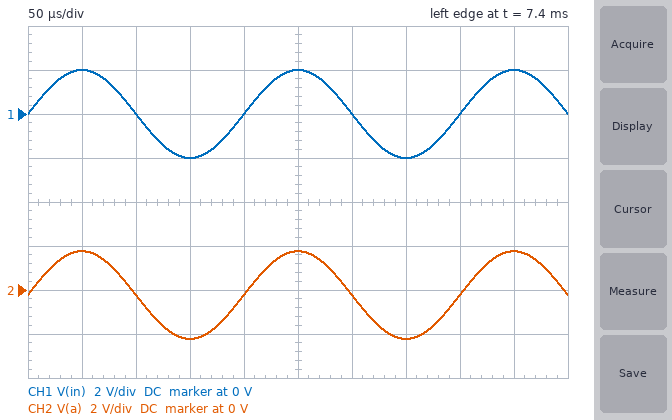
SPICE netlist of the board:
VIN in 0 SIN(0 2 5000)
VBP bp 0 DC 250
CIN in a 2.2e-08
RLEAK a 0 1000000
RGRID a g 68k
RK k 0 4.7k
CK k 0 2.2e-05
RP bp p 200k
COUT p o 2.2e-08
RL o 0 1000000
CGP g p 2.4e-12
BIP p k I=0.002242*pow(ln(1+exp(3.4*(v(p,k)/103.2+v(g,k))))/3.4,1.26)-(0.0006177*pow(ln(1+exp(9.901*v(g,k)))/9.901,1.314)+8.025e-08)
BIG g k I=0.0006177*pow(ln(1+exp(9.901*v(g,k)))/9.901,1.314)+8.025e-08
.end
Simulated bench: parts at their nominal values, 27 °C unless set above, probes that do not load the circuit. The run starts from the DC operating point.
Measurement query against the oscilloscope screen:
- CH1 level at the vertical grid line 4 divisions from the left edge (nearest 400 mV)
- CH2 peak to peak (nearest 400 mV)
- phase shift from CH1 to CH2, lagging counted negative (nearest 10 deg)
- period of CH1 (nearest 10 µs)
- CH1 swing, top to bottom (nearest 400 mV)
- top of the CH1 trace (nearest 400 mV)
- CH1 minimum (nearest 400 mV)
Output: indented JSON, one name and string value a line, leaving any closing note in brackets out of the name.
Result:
{
  "CH1 level at the vertical grid line 4 divisions from the left edge": "0 V",
  "CH2 peak to peak": "4.0 V",
  "phase shift from CH1 to CH2, lagging counted negative": "0 deg",
  "period of CH1": "200 µs",
  "CH1 swing, top to bottom": "4.0 V",
  "top of the CH1 trace": "2.0 V",
  "CH1 minimum": "-2.0 V"
}
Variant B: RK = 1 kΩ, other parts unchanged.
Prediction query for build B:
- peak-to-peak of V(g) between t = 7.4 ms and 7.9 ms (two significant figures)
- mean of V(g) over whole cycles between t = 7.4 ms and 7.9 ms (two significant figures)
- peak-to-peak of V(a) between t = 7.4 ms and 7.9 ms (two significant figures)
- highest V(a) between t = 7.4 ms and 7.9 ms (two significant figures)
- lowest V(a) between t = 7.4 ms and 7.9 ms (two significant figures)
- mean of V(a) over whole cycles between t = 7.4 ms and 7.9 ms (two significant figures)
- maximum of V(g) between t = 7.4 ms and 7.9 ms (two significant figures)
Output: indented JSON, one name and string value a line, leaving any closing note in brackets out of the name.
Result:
{
  "peak-to-peak of V(g) between t = 7.4 ms and 7.9 ms": "3.4 V",
  "mean of V(g) over whole cycles between t = 7.4 ms and 7.9 ms": "-900 mV",
  "peak-to-peak of V(a) between t = 7.4 ms and 7.9 ms": "4.0 V",
  "highest V(a) between t = 7.4 ms and 7.9 ms": "1.2 V",
  "lowest V(a) between t = 7.4 ms and 7.9 ms": "-2.8 V",
  "mean of V(a) over whole cycles between t = 7.4 ms and 7.9 ms": "-790 mV",
  "maximum of V(g) between t = 7.4 ms and 7.9 ms": "570 mV"
}
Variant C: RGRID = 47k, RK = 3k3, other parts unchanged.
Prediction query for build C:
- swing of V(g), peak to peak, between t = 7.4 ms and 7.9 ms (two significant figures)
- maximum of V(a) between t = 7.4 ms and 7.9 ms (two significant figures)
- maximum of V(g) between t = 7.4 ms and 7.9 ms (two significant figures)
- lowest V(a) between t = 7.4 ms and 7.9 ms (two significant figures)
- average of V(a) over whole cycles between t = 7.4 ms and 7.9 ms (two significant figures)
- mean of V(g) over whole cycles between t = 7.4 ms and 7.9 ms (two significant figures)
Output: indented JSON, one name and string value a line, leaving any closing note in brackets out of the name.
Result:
{
  "swing of V(g), peak to peak, between t = 7.4 ms and 7.9 ms": "3.7 V",
  "maximum of V(a) between t = 7.4 ms and 7.9 ms": "1.6 V",
  "maximum of V(g) between t = 7.4 ms and 7.9 ms": "1.3 V",
  "lowest V(a) between t = 7.4 ms and 7.9 ms": "-2.4 V",
  "average of V(a) over whole cycles between t = 7.4 ms and 7.9 ms": "-410 mV",
  "mean of V(g) over whole cycles between t = 7.4 ms and 7.9 ms": "-450 mV"
}
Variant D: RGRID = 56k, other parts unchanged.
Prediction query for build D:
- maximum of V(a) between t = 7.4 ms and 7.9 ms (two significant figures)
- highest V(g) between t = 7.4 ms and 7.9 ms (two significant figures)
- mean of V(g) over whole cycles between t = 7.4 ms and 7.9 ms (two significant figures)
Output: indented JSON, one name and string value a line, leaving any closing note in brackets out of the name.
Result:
{
  "maximum of V(a) between t = 7.4 ms and 7.9 ms": "1.7 V",
  "highest V(g) between t = 7.4 ms and 7.9 ms": "1.5 V",
  "mean of V(g) over whole cycles between t = 7.4 ms and 7.9 ms": "-280 mV"
}
